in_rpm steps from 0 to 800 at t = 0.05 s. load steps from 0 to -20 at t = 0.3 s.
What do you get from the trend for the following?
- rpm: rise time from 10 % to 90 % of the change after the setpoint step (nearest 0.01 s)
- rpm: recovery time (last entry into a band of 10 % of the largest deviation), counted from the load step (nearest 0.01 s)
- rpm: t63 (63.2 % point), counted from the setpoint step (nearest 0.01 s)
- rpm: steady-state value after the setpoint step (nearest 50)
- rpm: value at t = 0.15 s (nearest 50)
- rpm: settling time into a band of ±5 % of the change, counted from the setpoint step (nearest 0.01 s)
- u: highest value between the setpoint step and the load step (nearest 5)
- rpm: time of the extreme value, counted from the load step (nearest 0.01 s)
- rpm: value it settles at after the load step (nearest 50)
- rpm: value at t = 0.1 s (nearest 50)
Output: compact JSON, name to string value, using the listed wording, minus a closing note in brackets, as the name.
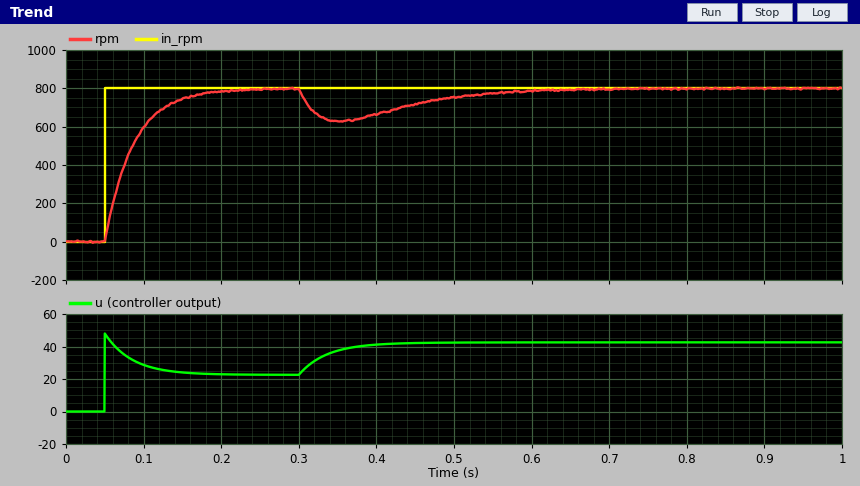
{"rpm: rise time from 10 % to 90 % of the change after the setpoint step": "0.08 s", "rpm: recovery time (last entry into a band of 10 % of the largest deviation), counted from the load step": "0.29 s", "rpm: t63 (63.2 % point), counted from the setpoint step": "0.04 s", "rpm: steady-state value after the setpoint step": "800", "rpm: value at t = 0.15 s": "750", "rpm: settling time into a band of ±5 % of the change, counted from the setpoint step": "0.11 s", "u: highest value between the setpoint step and the load step": "50", "rpm: time of the extreme value, counted from the load step": "0.05 s", "rpm: value it settles at after the load step": "800", "rpm: value at t = 0.1 s": "600"}
